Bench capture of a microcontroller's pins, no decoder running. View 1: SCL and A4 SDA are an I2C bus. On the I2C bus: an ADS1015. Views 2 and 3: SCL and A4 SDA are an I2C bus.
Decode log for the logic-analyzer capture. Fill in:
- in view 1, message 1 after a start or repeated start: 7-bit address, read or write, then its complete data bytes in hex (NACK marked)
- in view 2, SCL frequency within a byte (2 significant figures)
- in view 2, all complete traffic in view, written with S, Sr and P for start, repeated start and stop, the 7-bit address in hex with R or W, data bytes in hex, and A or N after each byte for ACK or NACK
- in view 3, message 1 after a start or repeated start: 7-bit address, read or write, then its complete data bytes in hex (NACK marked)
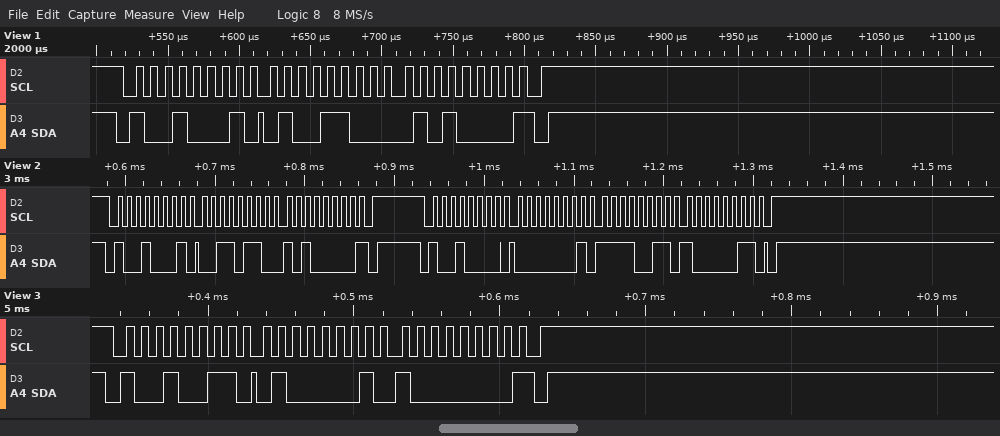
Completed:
0x48 read: 4C 50 NACK
100 kHz
S 48R A 36 A A0 N P S 48W A 01 A F3 A 83 A P
0x49 read: 41 80 NACK
